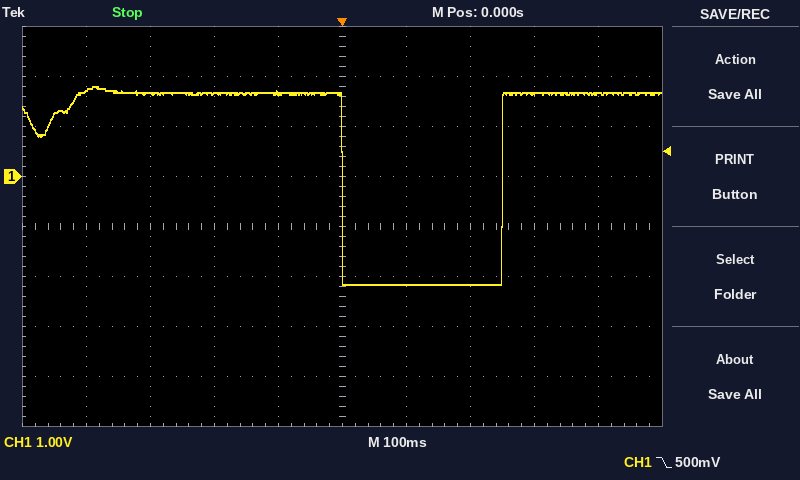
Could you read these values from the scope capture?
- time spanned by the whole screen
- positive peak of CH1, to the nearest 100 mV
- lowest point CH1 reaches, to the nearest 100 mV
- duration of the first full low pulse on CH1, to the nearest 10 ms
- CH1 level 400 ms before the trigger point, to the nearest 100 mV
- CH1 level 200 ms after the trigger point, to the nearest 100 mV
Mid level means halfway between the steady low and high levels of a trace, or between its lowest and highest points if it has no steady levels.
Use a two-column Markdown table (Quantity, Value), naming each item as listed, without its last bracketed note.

| Quantity | Value |
|---|---|
| time spanned by the whole screen | 1 s |
| positive peak of CH1, to the nearest 100 mV | 1.8 V |
| lowest point CH1 reaches, to the nearest 100 mV | -2.2 V |
| duration of the first full low pulse on CH1, to the nearest 10 ms | 250 ms |
| CH1 level 400 ms before the trigger point, to the nearest 100 mV | 1.7 V |
| CH1 level 200 ms after the trigger point, to the nearest 100 mV | -2.2 V |
